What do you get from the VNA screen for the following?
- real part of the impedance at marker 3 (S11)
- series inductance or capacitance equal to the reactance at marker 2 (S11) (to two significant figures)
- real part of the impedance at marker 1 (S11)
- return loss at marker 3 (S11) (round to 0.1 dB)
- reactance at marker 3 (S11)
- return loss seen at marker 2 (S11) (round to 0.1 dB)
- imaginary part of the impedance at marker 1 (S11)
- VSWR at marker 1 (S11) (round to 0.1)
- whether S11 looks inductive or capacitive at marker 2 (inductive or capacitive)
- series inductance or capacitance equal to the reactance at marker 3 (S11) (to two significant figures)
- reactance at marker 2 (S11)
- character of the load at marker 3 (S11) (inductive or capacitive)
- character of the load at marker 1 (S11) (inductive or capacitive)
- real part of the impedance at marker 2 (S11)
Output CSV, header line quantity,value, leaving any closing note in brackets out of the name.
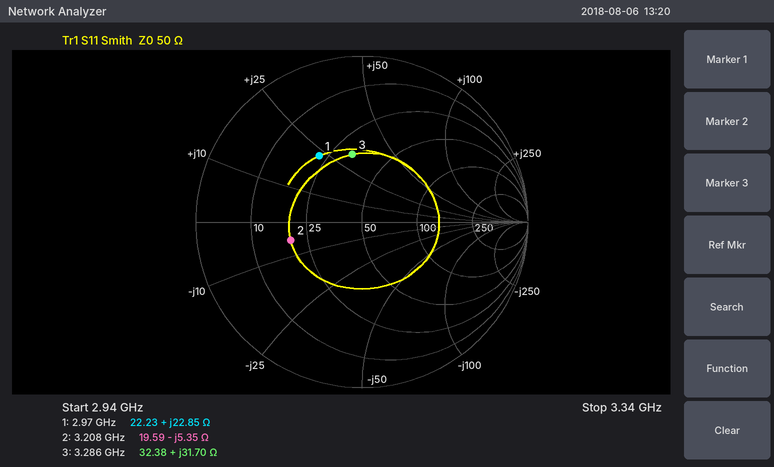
quantity,value
real part of the impedance at marker 3,32.38 Ω
series inductance or capacitance equal to the reactance at marker 2 (S11),9.3 pF
real part of the impedance at marker 1,22.23 Ω
return loss at marker 3 (S11),7.7 dB
reactance at marker 3,+31.70 Ω
return loss seen at marker 2 (S11),7.1 dB
imaginary part of the impedance at marker 1,+22.85 Ω
VSWR at marker 1 (S11),2.8
whether S11 looks inductive or capacitive at marker 2,capacitive
series inductance or capacitance equal to the reactance at marker 3 (S11),1.5 nH
reactance at marker 2,-5.35 Ω
character of the load at marker 3 (S11),inductive
character of the load at marker 1 (S11),inductive
real part of the impedance at marker 2,19.59 Ω
